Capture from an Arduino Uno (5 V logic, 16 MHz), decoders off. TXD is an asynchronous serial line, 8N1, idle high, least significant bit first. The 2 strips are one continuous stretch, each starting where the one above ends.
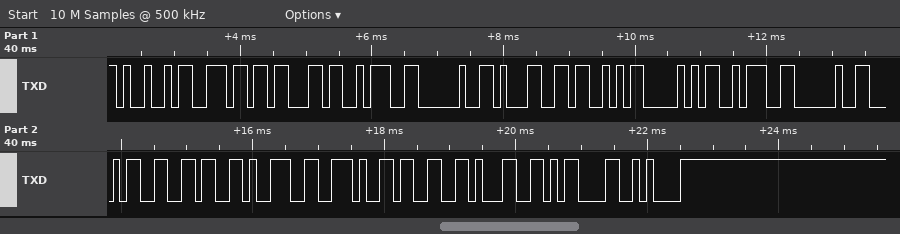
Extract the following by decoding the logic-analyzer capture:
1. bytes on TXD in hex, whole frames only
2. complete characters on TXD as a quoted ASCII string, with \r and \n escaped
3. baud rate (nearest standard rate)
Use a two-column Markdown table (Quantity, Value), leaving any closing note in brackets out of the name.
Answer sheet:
| Quantity | Value |
|---|---|
| bytes on TXD in hex, whole frames only | 49 6E 63 3A 20 31 53 50 3A 20 34 36 39 2E 33 31 0D 0A |
| complete characters on TXD as a quoted ASCII string, with \r and \n escaped | "Inc: 1SP: 469.31\r\n" |
| baud rate | 9600 baud |
